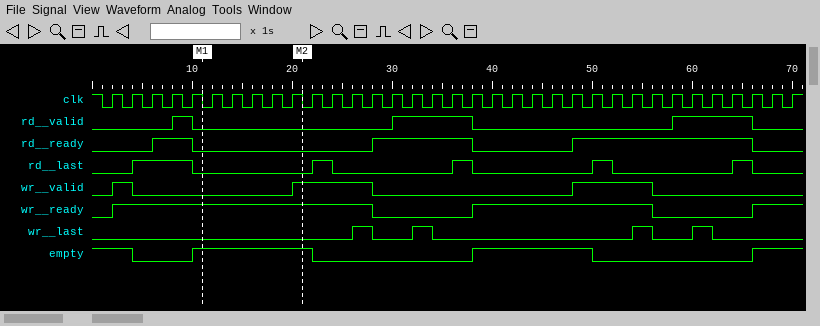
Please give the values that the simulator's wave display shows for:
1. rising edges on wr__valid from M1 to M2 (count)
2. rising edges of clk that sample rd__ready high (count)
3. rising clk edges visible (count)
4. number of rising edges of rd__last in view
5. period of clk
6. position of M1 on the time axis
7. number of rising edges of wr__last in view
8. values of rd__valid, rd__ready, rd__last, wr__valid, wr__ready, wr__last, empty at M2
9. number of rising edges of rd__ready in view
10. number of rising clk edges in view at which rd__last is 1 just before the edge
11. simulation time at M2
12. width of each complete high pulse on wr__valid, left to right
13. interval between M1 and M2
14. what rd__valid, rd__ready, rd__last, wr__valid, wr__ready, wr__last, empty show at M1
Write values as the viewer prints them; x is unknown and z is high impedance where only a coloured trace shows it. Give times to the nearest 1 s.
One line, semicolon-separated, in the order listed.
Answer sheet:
1; 16; 35; 5; 2 s; 11 s; 4; rd__valid=0, rd__ready=0, rd__last=0, wr__valid=1, wr__ready=1, wr__last=0, empty=1; 3; 7; 21 s; 2 s, 8 s, 8 s; 10 s; rd__valid=0, rd__ready=0, rd__last=0, wr__valid=0, wr__ready=1, wr__last=0, empty=1
